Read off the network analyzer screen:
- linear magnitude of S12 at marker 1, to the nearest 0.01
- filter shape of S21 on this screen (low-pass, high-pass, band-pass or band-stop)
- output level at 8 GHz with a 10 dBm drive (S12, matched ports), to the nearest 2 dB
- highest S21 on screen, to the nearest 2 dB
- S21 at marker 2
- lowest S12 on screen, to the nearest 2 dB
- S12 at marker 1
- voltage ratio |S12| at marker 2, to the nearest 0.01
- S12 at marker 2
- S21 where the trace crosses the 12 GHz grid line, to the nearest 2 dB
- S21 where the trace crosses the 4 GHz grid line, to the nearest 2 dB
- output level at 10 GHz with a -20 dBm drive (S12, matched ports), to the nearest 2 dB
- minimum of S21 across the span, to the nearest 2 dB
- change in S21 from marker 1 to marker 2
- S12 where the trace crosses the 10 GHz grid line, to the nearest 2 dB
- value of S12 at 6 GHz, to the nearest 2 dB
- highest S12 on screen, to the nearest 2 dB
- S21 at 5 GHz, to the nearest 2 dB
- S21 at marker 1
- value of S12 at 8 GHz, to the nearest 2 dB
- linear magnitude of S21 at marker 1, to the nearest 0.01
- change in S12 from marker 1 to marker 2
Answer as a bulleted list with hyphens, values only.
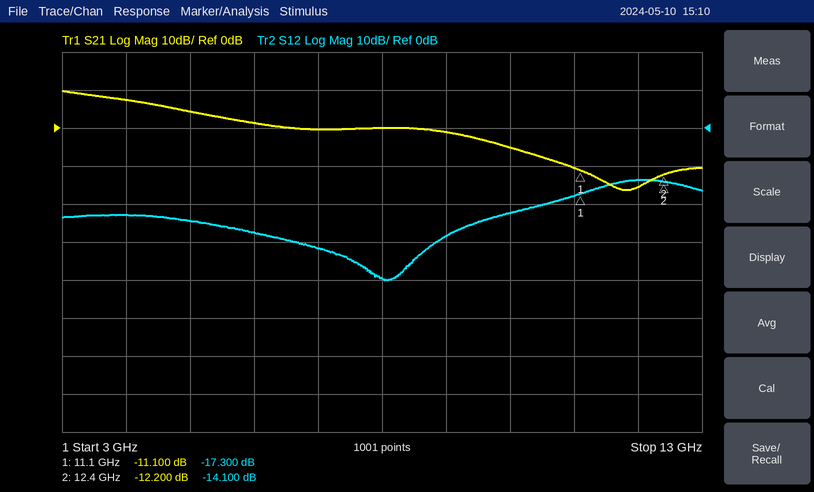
- 0.14
- low-pass
- -30 dBm
- 10 dB
- -12.200 dB
- -40 dB
- -17.300 dB
- 0.20
- -14.100 dB
- -16 dB
- 8 dB
- -42 dBm
- -16 dB
- -1.100 dB
- -22 dB
- -28 dB
- -14 dB
- 4 dB
- -11.100 dB
- -40 dB
- 0.28
- 3.200 dB
